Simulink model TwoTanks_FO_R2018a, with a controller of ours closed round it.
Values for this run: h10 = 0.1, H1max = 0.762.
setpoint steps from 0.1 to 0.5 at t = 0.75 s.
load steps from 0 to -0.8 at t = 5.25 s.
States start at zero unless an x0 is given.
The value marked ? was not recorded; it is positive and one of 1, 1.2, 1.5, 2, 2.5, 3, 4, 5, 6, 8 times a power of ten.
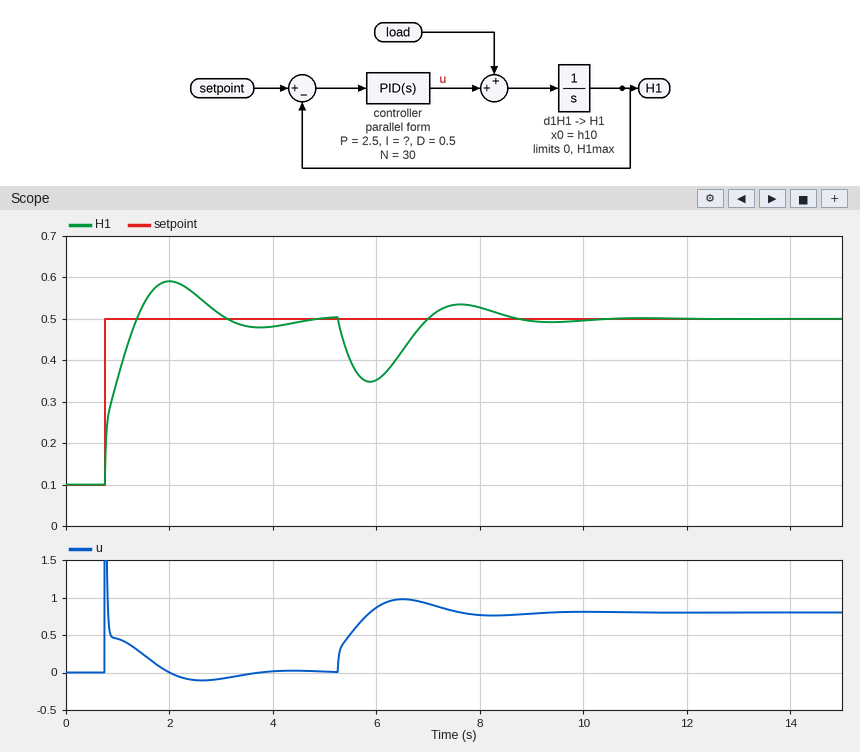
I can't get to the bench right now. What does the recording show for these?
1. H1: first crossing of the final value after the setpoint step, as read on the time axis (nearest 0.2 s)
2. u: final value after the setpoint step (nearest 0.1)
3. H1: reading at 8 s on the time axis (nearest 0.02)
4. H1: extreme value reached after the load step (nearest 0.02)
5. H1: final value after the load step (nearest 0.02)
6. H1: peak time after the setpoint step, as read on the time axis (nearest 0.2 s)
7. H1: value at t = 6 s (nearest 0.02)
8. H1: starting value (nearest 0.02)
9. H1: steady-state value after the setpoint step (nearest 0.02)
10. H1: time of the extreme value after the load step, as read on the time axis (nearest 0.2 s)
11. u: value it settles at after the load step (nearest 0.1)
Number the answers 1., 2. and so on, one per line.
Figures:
1. 1.4 s
2. 0.0
3. 0.52
4. 0.34
5. 0.50
6. 2.0 s
7. 0.36
8. 0.10
9. 0.50
10. 5.8 s
11. 0.8
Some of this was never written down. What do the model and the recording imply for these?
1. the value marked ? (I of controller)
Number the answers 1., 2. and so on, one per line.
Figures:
1. 6
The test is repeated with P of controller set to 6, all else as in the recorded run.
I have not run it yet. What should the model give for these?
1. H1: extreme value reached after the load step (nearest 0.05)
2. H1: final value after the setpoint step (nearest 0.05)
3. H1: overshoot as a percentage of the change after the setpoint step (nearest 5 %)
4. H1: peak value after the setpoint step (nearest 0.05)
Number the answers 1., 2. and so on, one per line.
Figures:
1. 0.40
2. 0.50
3. 10 %
4. 0.55
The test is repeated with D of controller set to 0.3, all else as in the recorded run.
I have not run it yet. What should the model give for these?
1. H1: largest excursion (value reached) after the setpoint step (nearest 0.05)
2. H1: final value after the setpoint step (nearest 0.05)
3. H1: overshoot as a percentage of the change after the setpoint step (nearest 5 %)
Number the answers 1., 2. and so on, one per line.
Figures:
1. 0.60
2. 0.50
3. 25 %
